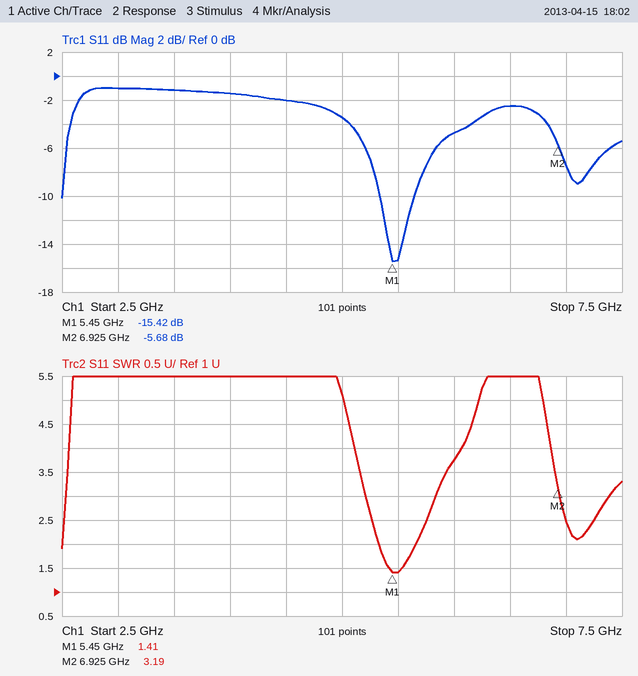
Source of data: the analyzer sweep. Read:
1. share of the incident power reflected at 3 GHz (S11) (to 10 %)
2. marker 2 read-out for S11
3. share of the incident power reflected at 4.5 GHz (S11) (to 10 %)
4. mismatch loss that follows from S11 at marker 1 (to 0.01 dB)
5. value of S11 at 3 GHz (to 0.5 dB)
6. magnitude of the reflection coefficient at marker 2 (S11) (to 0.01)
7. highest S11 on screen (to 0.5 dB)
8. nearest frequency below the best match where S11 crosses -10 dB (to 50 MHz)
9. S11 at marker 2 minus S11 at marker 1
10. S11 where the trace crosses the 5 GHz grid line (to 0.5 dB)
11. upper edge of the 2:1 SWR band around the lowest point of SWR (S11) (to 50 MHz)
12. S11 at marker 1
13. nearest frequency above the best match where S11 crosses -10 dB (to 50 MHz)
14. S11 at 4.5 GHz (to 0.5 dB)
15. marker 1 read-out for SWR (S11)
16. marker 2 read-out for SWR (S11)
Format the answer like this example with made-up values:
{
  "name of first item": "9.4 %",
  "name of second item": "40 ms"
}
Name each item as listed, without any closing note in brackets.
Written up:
{
  "share of the incident power reflected at 3 GHz (S11)": "80 %",
  "marker 2 read-out for S11": "-5.68 dB",
  "share of the incident power reflected at 4.5 GHz (S11)": "60 %",
  "mismatch loss that follows from S11 at marker 1": "0.13 dB",
  "value of S11 at 3 GHz": "-1.0 dB",
  "magnitude of the reflection coefficient at marker 2 (S11)": "0.52",
  "highest S11 on screen": "-1.0 dB",
  "nearest frequency below the best match where S11 crosses -10 dB": "5.35 GHz",
  "S11 at marker 2 minus S11 at marker 1": "9.74 dB",
  "S11 where the trace crosses the 5 GHz grid line": "-3.5 dB",
  "upper edge of the 2:1 SWR band around the lowest point of SWR (S11)": "5.65 GHz",
  "S11 at marker 1": "-15.42 dB",
  "nearest frequency above the best match where S11 crosses -10 dB": "5.65 GHz",
  "S11 at 4.5 GHz": "-2.0 dB",
  "marker 1 read-out for SWR": "1.41",
  "marker 2 read-out for SWR": "3.19"
}
